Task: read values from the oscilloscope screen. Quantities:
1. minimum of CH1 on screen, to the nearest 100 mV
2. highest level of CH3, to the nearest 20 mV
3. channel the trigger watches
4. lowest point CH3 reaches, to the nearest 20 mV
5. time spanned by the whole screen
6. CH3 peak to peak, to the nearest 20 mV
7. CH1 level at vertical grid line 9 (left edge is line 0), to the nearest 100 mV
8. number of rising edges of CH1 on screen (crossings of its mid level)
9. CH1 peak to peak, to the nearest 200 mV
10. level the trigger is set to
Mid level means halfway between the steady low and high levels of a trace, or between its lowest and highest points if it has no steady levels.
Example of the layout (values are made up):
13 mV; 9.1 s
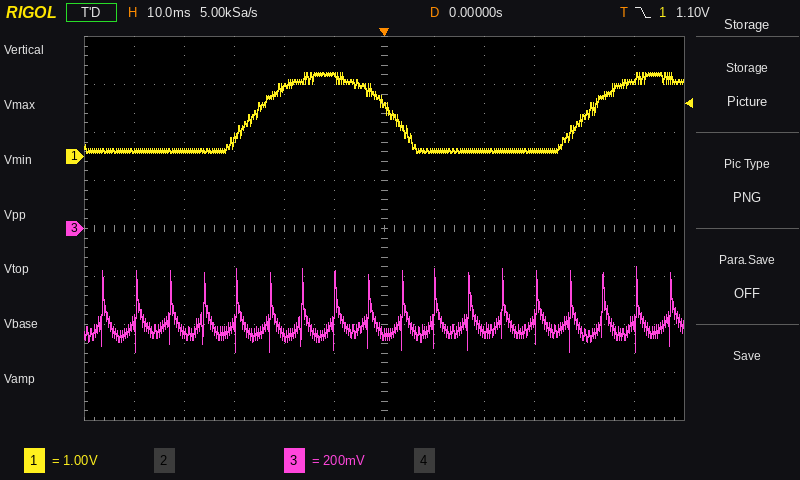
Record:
100 mV; -160 mV; CH1; -520 mV; 120 ms; 360 mV; 100 mV; 2; 1.6 V; 1.10 V
